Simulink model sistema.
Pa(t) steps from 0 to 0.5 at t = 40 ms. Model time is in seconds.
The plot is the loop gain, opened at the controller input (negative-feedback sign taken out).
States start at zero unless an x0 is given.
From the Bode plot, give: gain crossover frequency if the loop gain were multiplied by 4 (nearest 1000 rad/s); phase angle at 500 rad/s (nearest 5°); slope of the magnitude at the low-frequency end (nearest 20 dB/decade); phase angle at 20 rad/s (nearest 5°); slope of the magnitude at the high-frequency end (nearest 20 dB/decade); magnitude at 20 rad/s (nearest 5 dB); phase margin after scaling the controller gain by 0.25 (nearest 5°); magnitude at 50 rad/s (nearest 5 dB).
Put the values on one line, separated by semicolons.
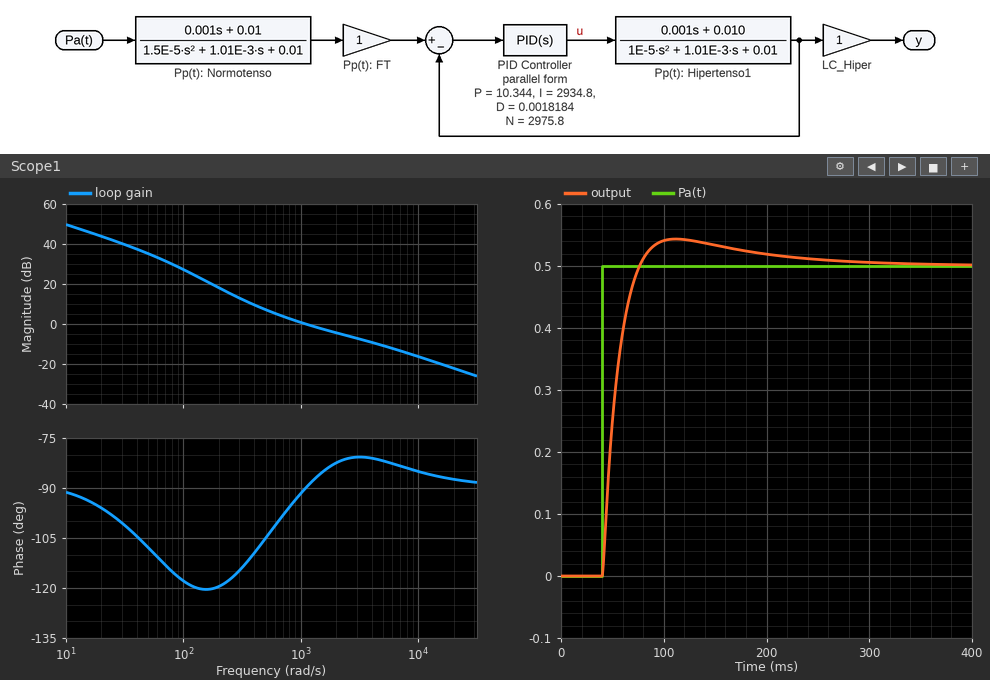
6000 rad/s; -105°; -20 dB/decade; -95°; -20 dB/decade; 45 dB; 65°; 35 dB
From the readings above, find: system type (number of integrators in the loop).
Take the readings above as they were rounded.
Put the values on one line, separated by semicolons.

1
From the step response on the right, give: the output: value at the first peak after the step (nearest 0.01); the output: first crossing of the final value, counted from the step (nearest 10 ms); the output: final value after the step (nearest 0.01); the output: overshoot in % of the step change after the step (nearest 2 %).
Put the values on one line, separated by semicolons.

0.54; 40 ms; 0.50; 8 %
